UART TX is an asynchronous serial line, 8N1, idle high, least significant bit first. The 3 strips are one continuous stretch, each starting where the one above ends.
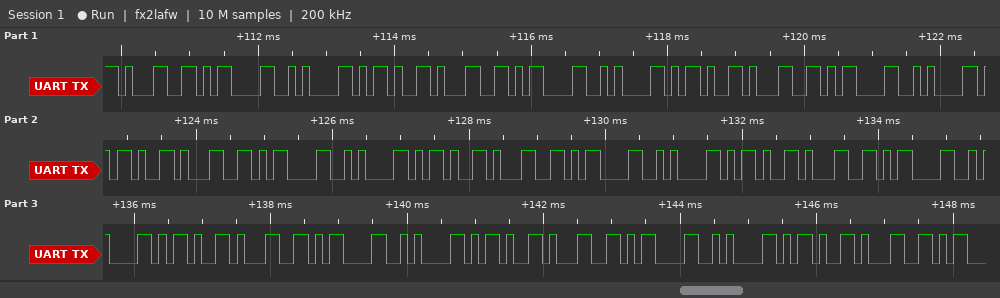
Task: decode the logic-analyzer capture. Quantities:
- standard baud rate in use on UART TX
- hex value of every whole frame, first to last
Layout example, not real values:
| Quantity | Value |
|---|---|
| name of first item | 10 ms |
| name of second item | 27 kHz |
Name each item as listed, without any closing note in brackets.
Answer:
| Quantity | Value |
|---|---|
| standard baud rate in use on UART TX | 9600 baud |
| hex value of every whole frame, first to last | 31 0D 0A 2D 31 0D 0A 2D 31 0D 0A 2D 31 0D 0A 2D 31 0D 0A 2D 31 0D 0A 2D 31 0D 0A 2D 31 0D 0A 2D 31 |
